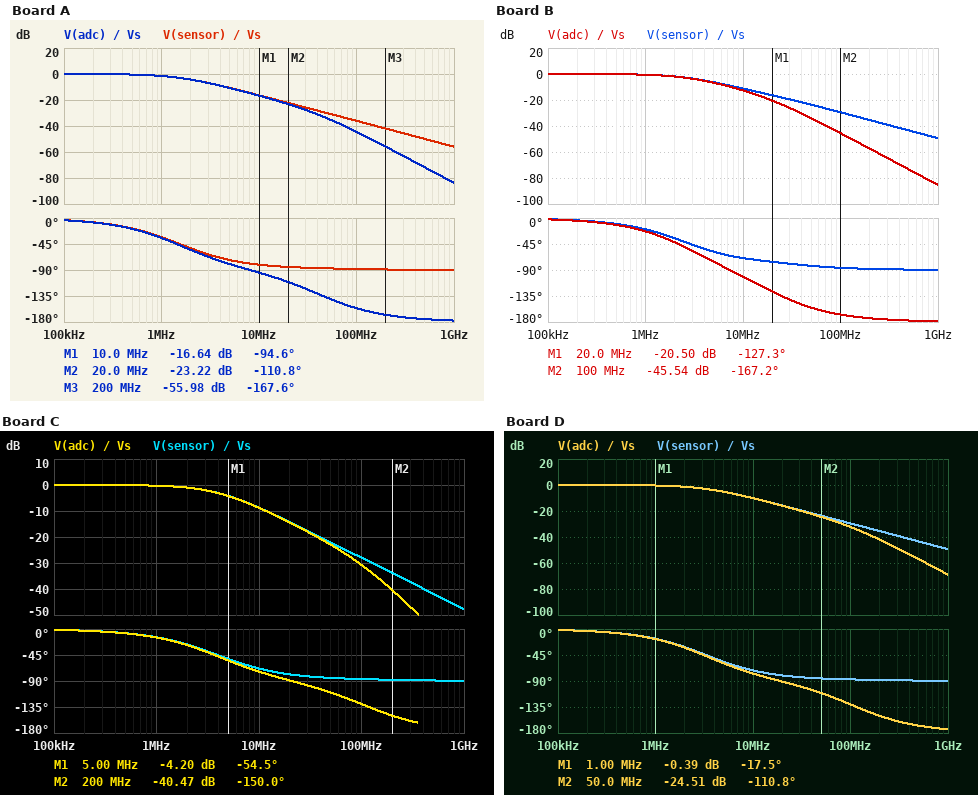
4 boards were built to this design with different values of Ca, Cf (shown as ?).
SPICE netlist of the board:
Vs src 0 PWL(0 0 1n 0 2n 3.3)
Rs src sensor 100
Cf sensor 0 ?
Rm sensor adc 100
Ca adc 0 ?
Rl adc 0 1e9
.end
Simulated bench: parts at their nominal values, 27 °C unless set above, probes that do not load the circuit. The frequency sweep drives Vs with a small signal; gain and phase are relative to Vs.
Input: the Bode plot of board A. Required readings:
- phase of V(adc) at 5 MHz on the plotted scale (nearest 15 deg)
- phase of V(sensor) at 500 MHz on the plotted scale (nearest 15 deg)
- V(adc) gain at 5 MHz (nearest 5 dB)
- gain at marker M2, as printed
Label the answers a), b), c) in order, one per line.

a) -75 deg
b) -90 deg
c) -10 dB
d) -23.22 dB
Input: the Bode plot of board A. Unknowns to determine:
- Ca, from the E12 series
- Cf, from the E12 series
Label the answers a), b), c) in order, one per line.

a) 39 pF
b) 1 nF
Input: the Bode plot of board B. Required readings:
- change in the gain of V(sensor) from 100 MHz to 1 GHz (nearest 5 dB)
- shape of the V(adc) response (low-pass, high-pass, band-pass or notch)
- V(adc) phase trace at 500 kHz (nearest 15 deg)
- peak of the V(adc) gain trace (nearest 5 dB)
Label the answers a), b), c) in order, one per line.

a) -20 dB
b) low-pass
c) -15 deg
d) 0 dB
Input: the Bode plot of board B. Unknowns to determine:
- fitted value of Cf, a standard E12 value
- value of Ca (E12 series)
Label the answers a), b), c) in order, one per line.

a) 470 pF
b) 100 pF
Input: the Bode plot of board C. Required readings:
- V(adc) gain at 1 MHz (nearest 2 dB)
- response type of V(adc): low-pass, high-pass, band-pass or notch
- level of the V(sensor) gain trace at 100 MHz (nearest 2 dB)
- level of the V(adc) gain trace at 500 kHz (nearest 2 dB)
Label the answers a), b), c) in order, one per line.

a) 0 dB
b) low-pass
c) -28 dB
d) 0 dB
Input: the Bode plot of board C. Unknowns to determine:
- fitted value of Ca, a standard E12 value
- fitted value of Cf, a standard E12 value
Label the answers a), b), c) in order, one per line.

a) 15 pF
b) 390 pF
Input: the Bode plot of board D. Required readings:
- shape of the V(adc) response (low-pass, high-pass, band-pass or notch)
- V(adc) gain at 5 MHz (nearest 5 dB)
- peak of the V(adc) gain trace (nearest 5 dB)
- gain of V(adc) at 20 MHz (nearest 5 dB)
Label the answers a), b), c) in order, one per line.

a) low-pass
b) -5 dB
c) 0 dB
d) -15 dB
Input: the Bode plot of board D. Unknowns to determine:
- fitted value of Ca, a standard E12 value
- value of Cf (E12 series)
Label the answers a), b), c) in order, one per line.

a) 15 pF
b) 470 pF
